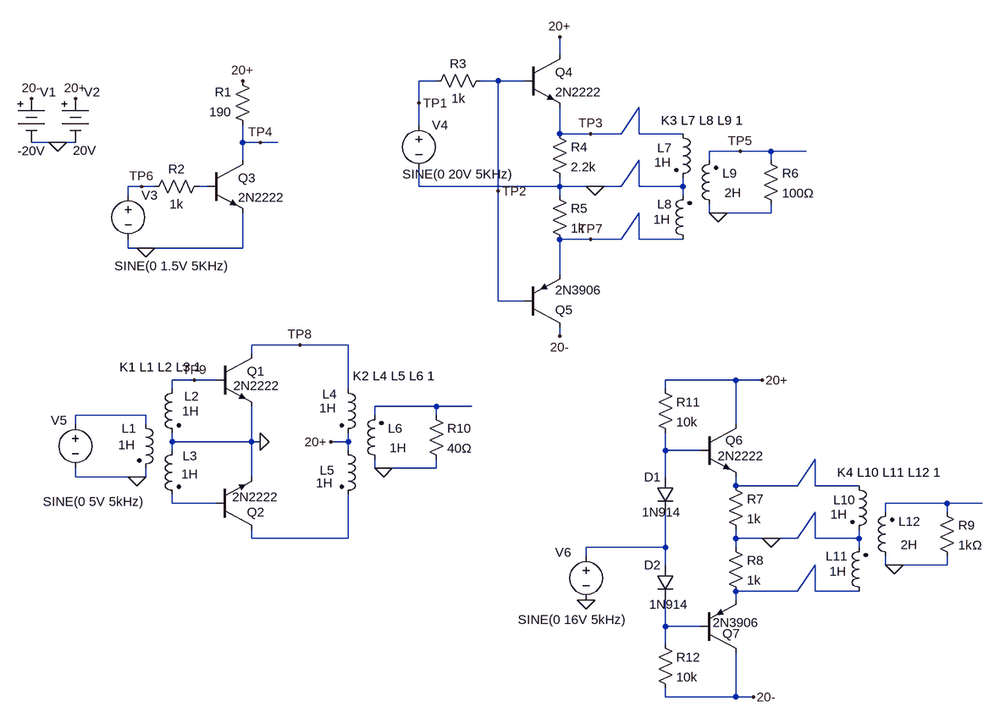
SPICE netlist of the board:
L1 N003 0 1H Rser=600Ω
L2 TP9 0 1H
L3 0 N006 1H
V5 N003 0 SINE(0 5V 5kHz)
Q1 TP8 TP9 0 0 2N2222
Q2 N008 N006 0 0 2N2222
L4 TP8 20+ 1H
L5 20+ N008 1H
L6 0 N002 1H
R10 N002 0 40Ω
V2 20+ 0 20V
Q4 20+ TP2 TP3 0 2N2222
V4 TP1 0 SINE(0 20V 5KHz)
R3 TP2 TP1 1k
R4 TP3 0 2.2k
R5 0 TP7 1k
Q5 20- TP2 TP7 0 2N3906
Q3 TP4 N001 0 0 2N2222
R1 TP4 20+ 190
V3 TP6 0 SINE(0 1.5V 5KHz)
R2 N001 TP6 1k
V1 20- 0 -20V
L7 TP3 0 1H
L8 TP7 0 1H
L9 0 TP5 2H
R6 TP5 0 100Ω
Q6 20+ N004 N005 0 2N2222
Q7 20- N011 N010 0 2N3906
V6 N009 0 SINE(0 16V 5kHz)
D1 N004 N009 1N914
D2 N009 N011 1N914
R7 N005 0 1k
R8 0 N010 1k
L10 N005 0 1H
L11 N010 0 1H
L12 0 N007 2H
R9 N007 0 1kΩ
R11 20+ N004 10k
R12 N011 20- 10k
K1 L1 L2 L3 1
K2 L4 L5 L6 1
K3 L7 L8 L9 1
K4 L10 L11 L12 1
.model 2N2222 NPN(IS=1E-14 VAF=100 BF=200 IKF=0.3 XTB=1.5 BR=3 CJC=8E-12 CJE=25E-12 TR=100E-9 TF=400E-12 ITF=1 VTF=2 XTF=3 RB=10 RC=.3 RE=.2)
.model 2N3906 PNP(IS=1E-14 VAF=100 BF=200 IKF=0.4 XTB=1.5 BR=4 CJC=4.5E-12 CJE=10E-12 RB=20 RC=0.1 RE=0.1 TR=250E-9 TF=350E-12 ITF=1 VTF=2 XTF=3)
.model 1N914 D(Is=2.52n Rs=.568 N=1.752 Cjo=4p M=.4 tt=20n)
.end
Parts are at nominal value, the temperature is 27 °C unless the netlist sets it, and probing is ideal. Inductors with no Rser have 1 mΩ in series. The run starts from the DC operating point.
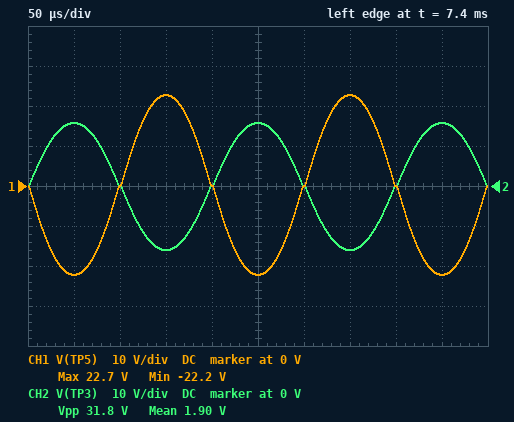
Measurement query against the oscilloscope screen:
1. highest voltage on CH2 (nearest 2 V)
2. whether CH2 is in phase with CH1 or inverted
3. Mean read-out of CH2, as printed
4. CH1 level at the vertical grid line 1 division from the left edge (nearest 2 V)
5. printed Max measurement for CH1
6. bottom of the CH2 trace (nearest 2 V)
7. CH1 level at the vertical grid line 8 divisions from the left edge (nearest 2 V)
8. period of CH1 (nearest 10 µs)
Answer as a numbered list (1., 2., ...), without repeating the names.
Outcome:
1. 16 V
2. inverted
3. 1.90 V
4. -22 V
5. 22.7 V
6. -16 V
7. 0 V
8. 200 µs
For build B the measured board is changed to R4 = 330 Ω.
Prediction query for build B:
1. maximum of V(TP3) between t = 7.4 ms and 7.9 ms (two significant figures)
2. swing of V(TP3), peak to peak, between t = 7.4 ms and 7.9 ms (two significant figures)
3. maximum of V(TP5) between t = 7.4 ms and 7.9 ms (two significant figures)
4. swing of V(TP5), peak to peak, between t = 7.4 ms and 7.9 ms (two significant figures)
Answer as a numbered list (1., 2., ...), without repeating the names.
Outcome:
1. 15 V
2. 31 V
3. 22 V
4. 44 V
